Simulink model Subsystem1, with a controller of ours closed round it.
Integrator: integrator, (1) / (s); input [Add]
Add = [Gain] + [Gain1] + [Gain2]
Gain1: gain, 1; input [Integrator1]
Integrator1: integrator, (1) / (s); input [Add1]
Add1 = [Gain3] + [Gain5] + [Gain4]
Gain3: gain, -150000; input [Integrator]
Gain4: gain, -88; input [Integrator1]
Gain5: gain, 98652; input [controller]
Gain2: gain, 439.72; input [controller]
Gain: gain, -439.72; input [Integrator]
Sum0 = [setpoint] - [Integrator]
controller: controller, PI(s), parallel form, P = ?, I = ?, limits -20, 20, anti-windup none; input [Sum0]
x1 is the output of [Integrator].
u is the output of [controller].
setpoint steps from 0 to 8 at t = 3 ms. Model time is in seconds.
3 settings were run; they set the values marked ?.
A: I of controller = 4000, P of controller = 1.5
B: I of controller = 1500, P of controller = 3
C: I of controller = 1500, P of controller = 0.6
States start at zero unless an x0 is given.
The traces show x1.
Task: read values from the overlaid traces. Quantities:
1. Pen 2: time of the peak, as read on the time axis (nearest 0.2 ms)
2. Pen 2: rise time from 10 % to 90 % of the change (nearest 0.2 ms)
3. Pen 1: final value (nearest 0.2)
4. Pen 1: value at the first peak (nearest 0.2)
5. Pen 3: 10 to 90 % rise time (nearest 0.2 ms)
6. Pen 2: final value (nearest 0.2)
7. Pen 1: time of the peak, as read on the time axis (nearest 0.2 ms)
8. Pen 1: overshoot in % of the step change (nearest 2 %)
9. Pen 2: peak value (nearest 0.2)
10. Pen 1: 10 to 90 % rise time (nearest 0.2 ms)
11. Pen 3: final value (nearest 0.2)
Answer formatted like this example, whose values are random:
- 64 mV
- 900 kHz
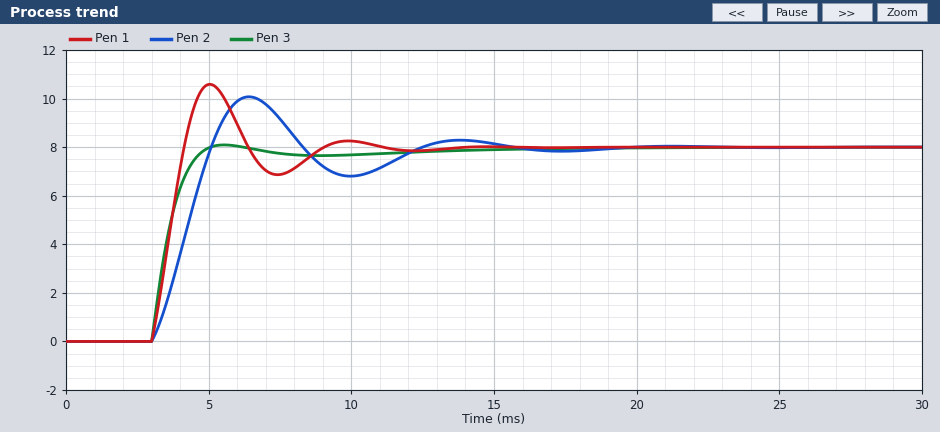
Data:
- 6.4 ms
- 1.6 ms
- 8.0
- 10.6
- 1.2 ms
- 8.0
- 5.0 ms
- 32 %
- 10.0
- 0.8 ms
- 8.0
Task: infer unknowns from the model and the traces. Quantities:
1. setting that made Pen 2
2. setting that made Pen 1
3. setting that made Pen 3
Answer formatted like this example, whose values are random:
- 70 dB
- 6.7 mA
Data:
- C
- A
- B
